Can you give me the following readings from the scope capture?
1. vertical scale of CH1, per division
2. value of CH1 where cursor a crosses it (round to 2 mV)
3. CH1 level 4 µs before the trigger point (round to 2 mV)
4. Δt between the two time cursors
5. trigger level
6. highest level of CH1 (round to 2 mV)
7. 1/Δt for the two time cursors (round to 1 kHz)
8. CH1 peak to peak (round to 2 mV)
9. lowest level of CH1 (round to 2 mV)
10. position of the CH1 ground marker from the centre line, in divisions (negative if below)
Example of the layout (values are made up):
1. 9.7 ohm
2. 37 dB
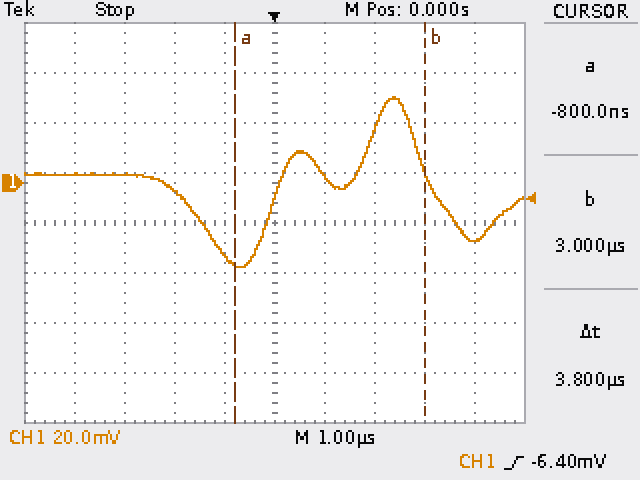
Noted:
1. 20 mV
2. -32 mV
3. 4 mV
4. 3.8 µs
5. -6.40 mV
6. 34 mV
7. 263 kHz
8. 68 mV
9. -34 mV
10. +0.8 div
